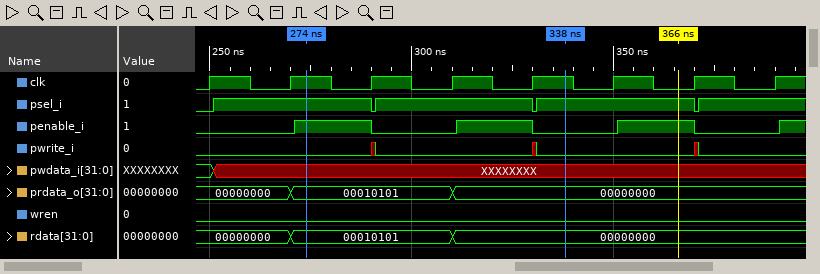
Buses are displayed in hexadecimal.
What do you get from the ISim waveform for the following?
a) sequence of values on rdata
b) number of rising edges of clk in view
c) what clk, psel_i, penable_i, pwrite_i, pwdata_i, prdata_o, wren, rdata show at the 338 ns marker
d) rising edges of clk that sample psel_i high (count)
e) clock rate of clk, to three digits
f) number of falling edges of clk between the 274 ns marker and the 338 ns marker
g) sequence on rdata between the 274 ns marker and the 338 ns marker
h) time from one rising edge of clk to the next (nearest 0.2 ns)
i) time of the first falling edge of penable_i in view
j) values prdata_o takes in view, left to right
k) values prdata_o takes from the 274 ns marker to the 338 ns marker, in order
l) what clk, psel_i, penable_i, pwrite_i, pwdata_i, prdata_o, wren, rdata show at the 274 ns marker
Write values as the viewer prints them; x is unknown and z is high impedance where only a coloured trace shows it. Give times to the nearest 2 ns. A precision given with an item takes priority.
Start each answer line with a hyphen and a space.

- 00000000, 00010101, 00000000
- 8
- clk=1, psel_i=1, penable_i=0, pwrite_i=0, pwdata_i=XXXXXXXX, prdata_o=00000000, wren=0, rdata=00000000
- 7
- 50.0 MHz
- 3
- 00010101, 00000000
- 20 ns
- 290 ns
- 00000000, 00010101, 00000000
- 00010101, 00000000
- clk=1, psel_i=1, penable_i=1, pwrite_i=0, pwdata_i=XXXXXXXX, prdata_o=00010101, wren=0, rdata=00010101
